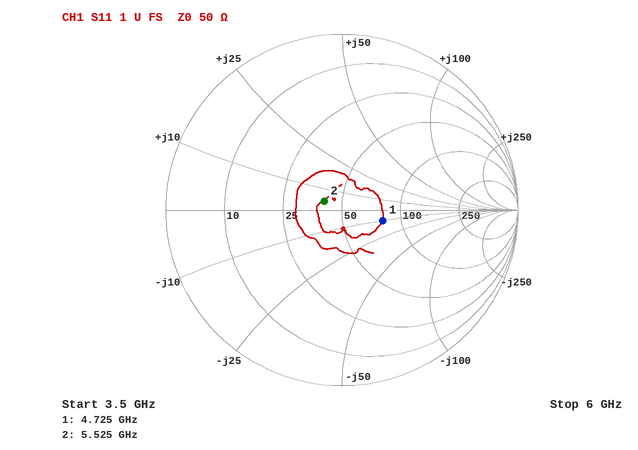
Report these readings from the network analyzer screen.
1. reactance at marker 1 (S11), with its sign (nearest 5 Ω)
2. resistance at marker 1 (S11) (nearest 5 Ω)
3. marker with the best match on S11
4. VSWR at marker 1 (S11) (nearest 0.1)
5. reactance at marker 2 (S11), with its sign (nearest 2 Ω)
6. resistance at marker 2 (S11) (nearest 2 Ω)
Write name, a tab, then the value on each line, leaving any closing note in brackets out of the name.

reactance at marker 1 (S11), with its sign	-10 Ω
resistance at marker 1 (S11)	80 Ω
marker with the best match on S11	marker 2
VSWR at marker 1 (S11)	1.6
reactance at marker 2 (S11), with its sign	+4 Ω
resistance at marker 2 (S11)	40 Ω
